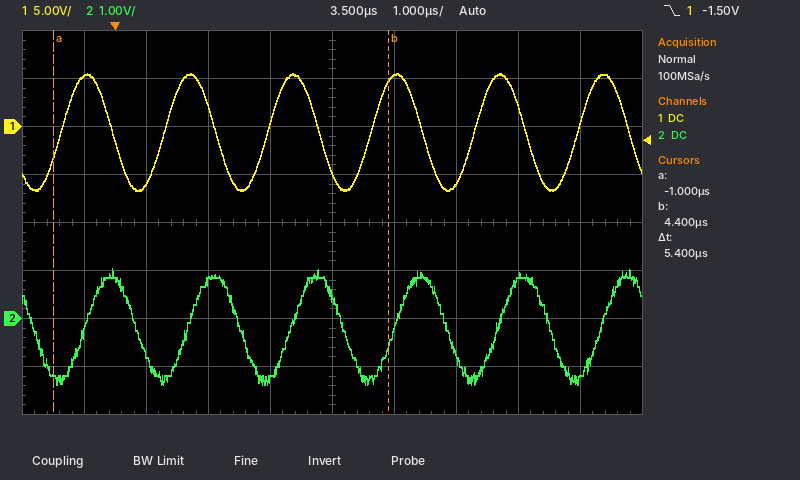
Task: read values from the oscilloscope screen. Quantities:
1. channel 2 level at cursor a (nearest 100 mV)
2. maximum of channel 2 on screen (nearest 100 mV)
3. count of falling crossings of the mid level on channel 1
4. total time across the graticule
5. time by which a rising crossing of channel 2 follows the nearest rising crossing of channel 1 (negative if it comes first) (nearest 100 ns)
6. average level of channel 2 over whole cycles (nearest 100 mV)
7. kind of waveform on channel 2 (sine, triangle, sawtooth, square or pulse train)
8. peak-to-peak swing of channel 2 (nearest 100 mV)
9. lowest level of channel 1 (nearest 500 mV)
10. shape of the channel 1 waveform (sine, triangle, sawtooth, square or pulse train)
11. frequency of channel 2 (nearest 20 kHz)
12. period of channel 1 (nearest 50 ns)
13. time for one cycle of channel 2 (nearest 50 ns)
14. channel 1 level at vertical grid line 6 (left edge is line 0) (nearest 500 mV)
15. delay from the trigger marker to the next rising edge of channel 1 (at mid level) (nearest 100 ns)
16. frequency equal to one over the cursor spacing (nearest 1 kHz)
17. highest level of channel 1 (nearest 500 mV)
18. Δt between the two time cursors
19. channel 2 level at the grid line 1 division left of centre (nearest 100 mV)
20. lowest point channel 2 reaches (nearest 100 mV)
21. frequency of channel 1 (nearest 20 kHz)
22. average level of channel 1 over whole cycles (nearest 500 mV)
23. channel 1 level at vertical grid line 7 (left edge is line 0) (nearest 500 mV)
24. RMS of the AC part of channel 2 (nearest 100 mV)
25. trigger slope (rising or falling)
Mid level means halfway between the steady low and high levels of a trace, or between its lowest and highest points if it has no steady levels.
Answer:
-1.3 V
1.0 V
6
10 µs
+400 ns
-200 mV
sine
2.4 V
-6.5 V
sine
600 kHz
1.65 µs
1.65 µs
5.5 V
800 ns
185 kHz
5.5 V
5.4 µs
-1.3 V
-1.4 V
600 kHz
-500 mV
-6.0 V
800 mV
falling
